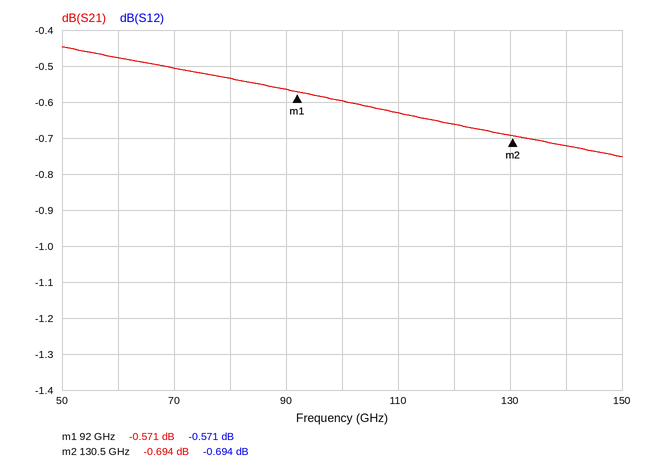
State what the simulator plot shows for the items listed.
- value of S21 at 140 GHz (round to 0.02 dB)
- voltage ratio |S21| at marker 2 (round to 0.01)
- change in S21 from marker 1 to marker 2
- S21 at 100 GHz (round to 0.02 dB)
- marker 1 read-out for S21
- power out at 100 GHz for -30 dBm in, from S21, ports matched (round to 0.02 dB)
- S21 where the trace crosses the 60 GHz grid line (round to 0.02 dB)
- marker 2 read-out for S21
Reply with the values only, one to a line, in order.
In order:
-0.72 dB
0.92
-0.123 dB
-0.60 dB
-0.571 dB
-30.60 dBm
-0.48 dB
-0.694 dB
